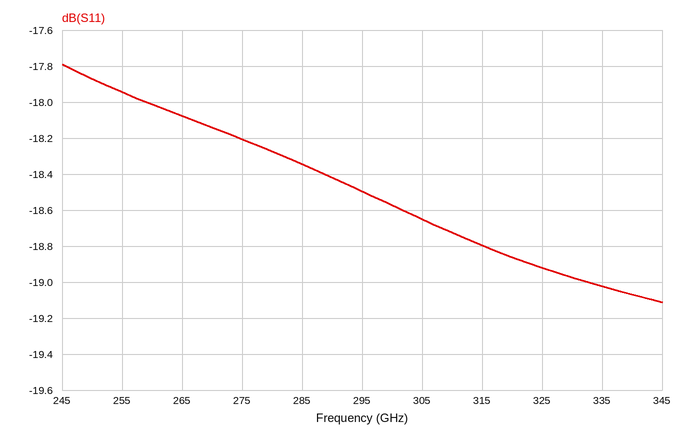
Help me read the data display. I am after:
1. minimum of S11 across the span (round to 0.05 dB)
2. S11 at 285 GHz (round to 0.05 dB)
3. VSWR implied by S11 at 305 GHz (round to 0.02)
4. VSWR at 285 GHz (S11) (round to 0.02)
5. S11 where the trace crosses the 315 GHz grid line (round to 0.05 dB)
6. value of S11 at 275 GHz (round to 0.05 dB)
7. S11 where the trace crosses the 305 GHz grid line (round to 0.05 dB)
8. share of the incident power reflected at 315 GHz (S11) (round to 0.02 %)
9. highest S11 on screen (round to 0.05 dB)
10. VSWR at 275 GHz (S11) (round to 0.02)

-19.10 dB
-18.35 dB
1.26
1.28
-18.80 dB
-18.20 dB
-18.65 dB
1.32 %
-17.80 dB
1.28
